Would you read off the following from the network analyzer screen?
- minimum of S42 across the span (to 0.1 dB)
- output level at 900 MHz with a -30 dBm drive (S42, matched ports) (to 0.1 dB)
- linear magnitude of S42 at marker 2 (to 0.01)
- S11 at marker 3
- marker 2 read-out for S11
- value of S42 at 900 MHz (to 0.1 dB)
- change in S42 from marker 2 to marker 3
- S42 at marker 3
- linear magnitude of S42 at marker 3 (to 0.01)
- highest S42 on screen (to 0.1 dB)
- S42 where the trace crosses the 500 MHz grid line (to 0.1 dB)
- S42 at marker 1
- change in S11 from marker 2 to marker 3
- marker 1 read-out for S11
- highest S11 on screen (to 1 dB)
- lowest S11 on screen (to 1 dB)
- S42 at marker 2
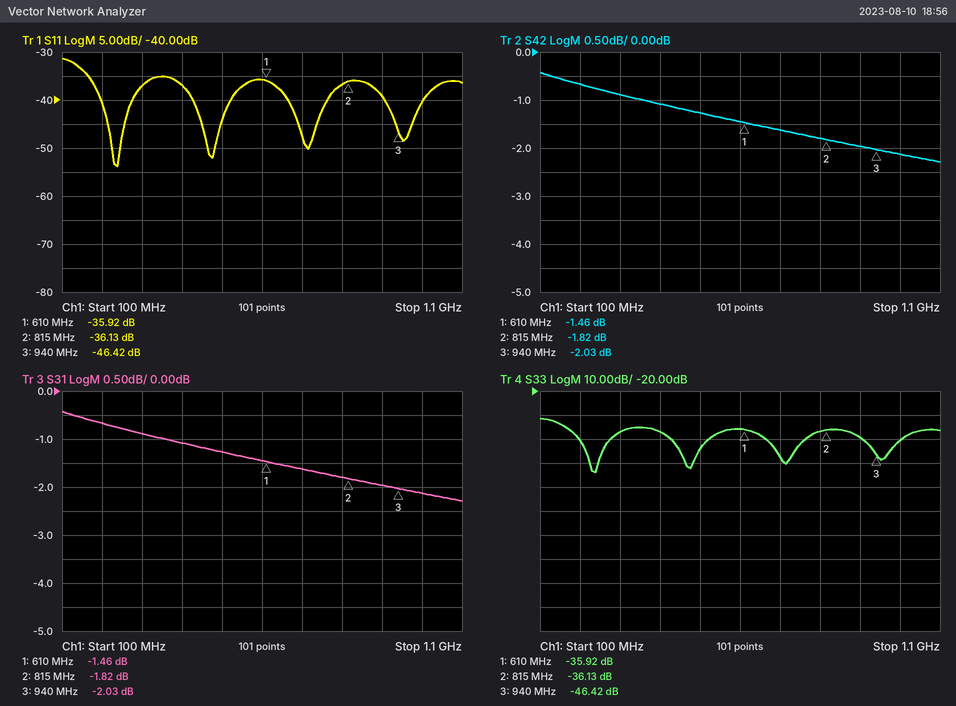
-2.3 dB
-32.0 dBm
0.81
-46.42 dB
-36.13 dB
-2.0 dB
-0.21 dB
-2.03 dB
0.79
-0.4 dB
-1.3 dB
-1.46 dB
-10.29 dB
-35.92 dB
-31 dB
-54 dB
-1.82 dB
